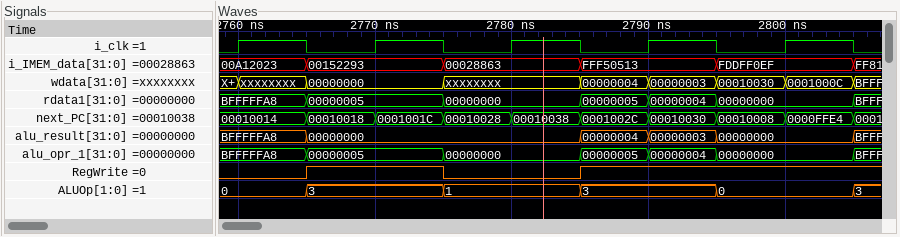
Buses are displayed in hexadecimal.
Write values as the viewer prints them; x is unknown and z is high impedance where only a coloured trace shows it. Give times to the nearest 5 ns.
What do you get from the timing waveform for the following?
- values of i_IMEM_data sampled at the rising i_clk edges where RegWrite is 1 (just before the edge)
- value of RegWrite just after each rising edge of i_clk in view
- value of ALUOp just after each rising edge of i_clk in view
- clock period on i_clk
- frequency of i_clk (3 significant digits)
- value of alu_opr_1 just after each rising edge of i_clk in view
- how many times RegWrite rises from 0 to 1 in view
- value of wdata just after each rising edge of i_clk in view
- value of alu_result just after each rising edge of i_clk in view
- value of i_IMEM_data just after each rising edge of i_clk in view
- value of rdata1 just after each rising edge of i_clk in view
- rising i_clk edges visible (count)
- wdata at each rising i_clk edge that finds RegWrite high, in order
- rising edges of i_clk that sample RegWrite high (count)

00152293, FFF50513, FDDFF0EF
0 1 0 1 1
0, 3, 1, 3, 0
10 ns
100 MHz
BFFFFFA8, 00000005, 00000000, 00000004, 00000000
2
xxxxxxxx, 00000000, xxxxxxxx, 00000003, 0001000C
BFFFFFA8, 00000000, 00000000, 00000003, 00000000
00A12023, 00152293, 00028863, FFF50513, FDDFF0EF
BFFFFFA8, 00000005, 00000000, 00000004, 00000000
5
00000000, 00000004, 00010030
3
